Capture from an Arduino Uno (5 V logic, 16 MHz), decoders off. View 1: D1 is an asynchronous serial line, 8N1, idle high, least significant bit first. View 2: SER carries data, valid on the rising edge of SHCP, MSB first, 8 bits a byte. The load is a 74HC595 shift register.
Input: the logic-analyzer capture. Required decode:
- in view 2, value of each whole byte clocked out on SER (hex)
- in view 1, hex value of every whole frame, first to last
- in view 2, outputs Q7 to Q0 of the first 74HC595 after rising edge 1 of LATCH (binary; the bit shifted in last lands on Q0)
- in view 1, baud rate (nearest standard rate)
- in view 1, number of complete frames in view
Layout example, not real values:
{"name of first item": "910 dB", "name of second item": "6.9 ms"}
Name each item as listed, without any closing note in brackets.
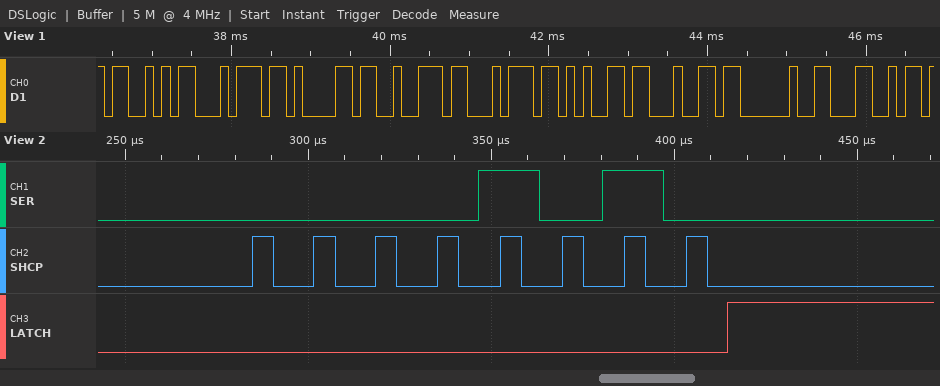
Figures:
{"in view 2, value of each whole byte clocked out on SER": "0A", "in view 1, hex value of every whole frame, first to last": "53 74 61 72 74 65 64 20 4C", "in view 2, outputs Q7 to Q0 of the first 74HC595 after rising edge 1 of LATCH": "00001010", "in view 1, baud rate": "9600 baud", "in view 1, number of complete frames in view": "9"}
